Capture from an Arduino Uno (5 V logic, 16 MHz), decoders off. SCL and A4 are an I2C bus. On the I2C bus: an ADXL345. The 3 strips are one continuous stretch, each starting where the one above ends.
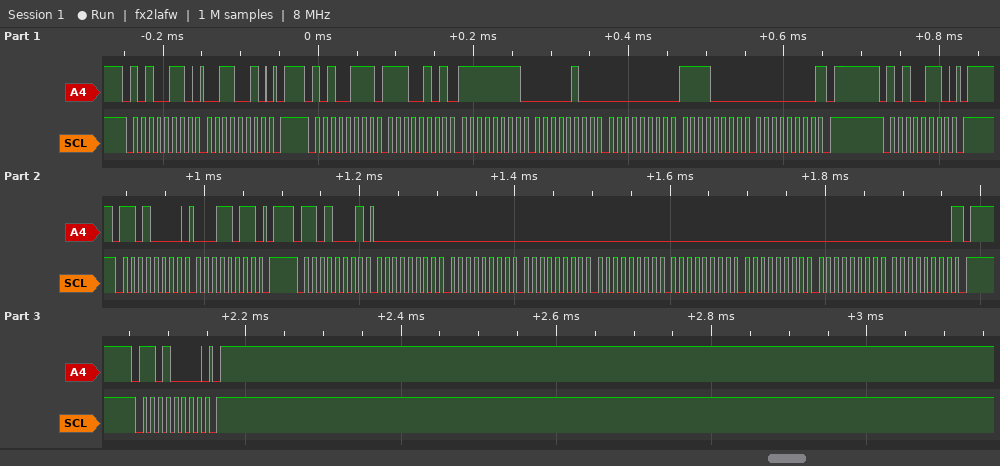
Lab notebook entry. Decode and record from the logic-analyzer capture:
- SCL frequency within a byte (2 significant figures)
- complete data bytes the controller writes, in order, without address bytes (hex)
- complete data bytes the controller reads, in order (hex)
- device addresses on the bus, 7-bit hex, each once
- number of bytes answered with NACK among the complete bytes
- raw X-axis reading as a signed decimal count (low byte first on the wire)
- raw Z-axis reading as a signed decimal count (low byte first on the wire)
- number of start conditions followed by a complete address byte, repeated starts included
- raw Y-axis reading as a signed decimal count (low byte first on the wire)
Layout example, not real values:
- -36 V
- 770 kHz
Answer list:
- 100 kHz
- 32 1B
- E5 FF 04 00 F0 00 00 00 00 00 00 00 00 00
- 0x53 0x68
- 2
- -27
- 240
- 6
- 4
